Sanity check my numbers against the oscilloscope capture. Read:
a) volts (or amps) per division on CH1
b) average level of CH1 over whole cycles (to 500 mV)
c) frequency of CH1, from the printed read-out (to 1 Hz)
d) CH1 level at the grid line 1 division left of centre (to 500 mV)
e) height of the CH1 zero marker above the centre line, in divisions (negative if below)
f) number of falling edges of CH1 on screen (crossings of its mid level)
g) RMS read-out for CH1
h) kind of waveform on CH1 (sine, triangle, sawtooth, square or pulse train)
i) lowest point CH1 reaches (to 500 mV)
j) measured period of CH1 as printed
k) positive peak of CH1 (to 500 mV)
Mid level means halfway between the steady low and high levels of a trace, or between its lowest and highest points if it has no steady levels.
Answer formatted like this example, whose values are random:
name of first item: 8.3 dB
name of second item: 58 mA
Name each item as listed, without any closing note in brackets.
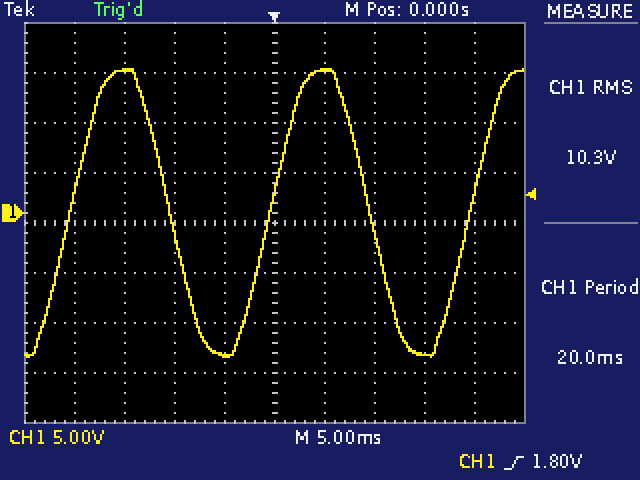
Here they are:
volts (or amps) per division on CH1: 5 V
average level of CH1 over whole cycles: 0.0 V
frequency of CH1, from the printed read-out: 50 Hz
CH1 level at the grid line 1 division left of centre: -14.0 V
height of the CH1 zero marker above the centre line, in divisions: +0.2 div
number of falling edges of CH1 on screen: 2
RMS read-out for CH1: 10.3 V
kind of waveform on CH1: sine
lowest point CH1 reaches: -14.5 V
measured period of CH1 as printed: 20.0 ms
positive peak of CH1: 14.5 V
